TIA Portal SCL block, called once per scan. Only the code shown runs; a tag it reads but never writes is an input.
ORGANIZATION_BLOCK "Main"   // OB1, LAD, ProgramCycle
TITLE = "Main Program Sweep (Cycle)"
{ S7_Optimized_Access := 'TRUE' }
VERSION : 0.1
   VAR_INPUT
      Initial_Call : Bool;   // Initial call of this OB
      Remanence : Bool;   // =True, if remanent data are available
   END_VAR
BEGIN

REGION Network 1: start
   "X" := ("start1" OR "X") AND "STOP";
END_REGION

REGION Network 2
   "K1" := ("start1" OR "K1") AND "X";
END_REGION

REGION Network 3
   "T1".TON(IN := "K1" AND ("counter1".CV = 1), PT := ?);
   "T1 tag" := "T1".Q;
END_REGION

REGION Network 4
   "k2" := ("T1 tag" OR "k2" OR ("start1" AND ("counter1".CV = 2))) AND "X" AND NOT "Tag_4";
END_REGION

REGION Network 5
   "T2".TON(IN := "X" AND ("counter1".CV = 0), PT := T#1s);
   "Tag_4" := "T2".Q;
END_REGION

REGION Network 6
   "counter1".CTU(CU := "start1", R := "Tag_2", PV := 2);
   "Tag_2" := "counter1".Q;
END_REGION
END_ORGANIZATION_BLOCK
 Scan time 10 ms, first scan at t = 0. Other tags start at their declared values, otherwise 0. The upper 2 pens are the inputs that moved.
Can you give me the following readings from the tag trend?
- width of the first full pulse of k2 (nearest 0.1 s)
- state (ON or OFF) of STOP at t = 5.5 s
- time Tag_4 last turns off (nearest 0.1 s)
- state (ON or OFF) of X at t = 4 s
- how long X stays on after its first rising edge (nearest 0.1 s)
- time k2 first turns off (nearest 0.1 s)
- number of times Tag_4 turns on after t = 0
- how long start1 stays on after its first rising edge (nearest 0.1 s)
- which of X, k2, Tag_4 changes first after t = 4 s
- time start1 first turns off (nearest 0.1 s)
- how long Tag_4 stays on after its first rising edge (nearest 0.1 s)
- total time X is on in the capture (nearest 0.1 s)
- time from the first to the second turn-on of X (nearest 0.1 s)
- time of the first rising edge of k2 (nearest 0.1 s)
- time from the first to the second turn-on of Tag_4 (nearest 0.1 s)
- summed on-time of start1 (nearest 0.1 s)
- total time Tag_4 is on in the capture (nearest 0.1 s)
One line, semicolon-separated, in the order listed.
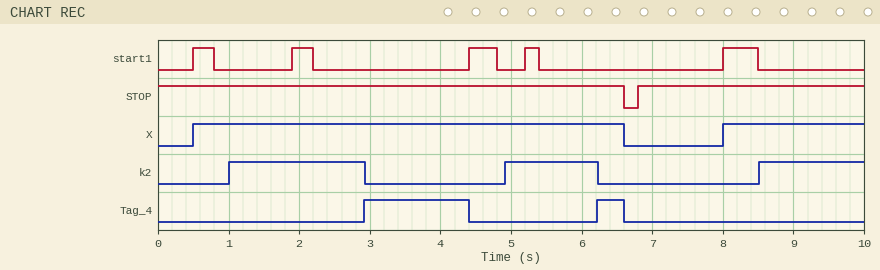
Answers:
1.9 s; ON; 6.6 s; ON; 6.1 s; 2.9 s; 2; 0.3 s; Tag_4; 0.8 s; 1.5 s; 8.1 s; 7.5 s; 1.0 s; 3.3 s; 1.7 s; 1.9 s
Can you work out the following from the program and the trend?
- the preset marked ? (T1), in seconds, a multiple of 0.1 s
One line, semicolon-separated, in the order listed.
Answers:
0.5 s
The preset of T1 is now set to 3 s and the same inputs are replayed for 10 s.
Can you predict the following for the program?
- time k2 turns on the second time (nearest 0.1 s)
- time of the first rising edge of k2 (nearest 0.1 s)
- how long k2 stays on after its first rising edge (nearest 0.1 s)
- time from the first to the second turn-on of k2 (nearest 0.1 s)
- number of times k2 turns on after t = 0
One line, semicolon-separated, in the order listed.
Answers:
5.2 s; 1.9 s; 1.0 s; 3.3 s; 2
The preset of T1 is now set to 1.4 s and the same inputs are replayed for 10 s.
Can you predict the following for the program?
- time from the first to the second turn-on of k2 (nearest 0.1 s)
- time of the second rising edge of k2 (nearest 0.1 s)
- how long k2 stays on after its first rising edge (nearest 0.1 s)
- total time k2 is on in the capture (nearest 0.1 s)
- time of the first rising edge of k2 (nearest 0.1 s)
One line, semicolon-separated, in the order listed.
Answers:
3.3 s; 5.2 s; 1.0 s; 2.6 s; 1.9 s
